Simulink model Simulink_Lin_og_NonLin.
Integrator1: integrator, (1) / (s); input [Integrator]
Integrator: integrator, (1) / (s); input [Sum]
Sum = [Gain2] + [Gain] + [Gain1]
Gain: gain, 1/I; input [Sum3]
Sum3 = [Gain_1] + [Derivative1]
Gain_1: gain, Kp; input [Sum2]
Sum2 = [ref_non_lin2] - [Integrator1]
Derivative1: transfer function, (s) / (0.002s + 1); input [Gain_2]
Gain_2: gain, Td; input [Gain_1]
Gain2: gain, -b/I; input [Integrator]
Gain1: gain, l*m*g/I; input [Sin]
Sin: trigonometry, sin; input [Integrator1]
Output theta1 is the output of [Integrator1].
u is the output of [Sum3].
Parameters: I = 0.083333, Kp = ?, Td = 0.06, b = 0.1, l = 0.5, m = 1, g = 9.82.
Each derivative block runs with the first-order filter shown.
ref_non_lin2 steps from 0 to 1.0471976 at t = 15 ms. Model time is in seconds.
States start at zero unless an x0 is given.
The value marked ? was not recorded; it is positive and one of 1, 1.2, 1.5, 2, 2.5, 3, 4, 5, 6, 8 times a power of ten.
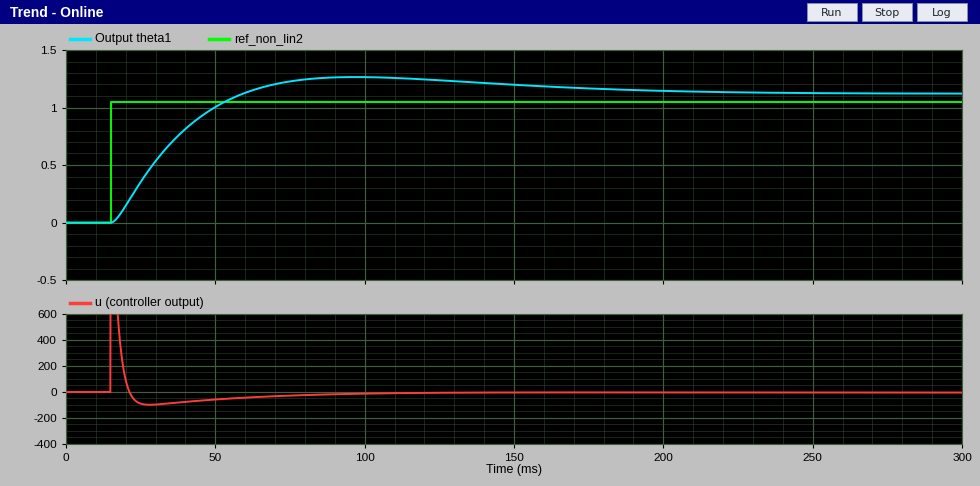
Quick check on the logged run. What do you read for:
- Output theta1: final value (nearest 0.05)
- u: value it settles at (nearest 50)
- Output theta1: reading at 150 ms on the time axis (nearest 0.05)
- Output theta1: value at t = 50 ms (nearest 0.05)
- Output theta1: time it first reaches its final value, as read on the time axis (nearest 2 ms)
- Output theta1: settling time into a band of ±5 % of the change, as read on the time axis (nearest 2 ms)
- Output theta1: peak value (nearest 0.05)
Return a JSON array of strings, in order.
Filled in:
["1.10", "0", "1.20", "1.00", "60 ms", "166 ms", "1.25"]
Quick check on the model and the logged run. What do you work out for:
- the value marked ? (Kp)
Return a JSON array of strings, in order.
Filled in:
["60"]
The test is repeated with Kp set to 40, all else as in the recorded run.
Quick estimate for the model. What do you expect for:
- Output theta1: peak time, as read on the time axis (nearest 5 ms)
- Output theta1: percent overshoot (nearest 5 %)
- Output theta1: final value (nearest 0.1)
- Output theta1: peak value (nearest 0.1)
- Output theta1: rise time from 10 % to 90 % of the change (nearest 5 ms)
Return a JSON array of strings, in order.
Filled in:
["125 ms", "15 %", "1.2", "1.3", "45 ms"]
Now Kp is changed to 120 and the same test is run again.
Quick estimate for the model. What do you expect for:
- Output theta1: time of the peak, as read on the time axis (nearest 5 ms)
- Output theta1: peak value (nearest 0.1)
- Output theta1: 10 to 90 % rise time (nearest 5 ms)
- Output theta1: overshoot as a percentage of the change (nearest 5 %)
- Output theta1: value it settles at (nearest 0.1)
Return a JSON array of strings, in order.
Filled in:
["60 ms", "1.2", "15 ms", "10 %", "1.1"]
